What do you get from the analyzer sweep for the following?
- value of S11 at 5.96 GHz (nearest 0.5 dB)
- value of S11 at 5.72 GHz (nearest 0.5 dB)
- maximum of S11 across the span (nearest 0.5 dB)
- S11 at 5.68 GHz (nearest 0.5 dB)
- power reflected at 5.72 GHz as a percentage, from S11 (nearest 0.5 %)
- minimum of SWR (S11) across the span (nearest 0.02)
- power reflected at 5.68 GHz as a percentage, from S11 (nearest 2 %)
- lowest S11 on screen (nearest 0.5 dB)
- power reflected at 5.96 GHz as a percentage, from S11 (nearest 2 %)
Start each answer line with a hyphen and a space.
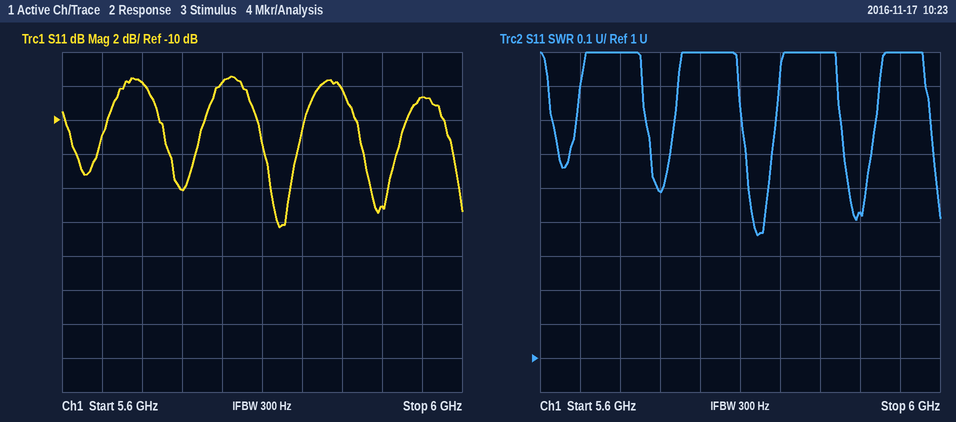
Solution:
- -8.5 dB
- -14.0 dB
- -7.5 dB
- -8.0 dB
- 4.0 %
- 1.36
- 16 %
- -16.5 dB
- 14 %
